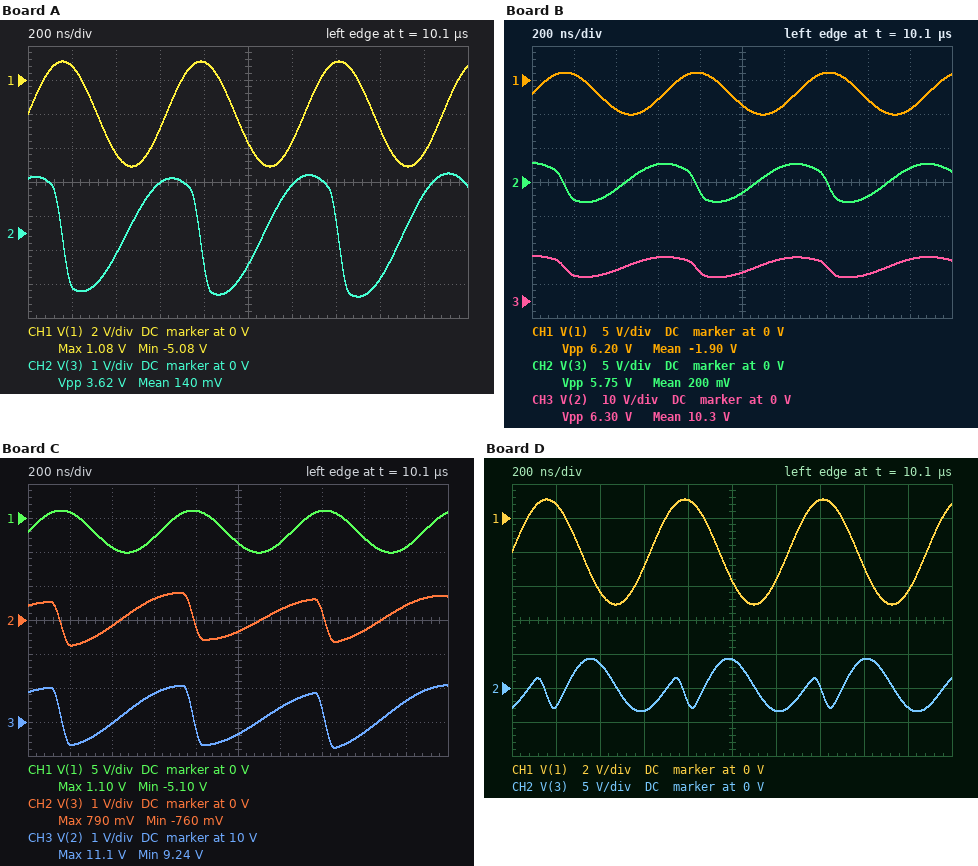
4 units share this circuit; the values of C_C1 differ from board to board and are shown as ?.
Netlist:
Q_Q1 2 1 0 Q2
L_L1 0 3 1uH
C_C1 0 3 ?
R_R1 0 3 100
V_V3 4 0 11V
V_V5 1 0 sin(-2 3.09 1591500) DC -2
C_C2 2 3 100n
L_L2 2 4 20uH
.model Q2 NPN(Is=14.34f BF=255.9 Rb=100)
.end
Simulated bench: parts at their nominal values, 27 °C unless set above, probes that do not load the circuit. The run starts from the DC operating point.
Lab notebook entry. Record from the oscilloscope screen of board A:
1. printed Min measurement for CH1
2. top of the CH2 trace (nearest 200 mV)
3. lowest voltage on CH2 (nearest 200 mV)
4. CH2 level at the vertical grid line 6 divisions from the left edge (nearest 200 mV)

-5.08 V
1.8 V
-1.8 V
1.4 V
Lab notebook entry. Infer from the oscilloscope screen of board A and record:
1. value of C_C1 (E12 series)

18 nF
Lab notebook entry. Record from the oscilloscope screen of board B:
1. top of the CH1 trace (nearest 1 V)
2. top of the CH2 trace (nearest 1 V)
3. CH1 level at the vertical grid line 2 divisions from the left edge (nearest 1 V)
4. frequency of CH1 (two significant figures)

1 V
3 V
-4 V
1.6 MHz
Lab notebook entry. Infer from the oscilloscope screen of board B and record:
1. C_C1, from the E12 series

15 nF
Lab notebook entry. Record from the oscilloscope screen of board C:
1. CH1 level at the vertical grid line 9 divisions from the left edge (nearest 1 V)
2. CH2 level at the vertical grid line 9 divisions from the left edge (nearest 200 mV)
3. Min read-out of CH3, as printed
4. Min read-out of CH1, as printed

-4 V
400 mV
9.24 V
-5.10 V
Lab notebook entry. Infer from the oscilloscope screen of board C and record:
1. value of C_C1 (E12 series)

33 nF
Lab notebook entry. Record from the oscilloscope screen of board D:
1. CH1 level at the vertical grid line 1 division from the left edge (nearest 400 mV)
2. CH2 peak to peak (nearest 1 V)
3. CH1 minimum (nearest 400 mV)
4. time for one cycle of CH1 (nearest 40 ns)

800 mV
8 V
-5.2 V
640 ns
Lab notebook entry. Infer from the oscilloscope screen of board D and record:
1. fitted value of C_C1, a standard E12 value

5.6 nF
